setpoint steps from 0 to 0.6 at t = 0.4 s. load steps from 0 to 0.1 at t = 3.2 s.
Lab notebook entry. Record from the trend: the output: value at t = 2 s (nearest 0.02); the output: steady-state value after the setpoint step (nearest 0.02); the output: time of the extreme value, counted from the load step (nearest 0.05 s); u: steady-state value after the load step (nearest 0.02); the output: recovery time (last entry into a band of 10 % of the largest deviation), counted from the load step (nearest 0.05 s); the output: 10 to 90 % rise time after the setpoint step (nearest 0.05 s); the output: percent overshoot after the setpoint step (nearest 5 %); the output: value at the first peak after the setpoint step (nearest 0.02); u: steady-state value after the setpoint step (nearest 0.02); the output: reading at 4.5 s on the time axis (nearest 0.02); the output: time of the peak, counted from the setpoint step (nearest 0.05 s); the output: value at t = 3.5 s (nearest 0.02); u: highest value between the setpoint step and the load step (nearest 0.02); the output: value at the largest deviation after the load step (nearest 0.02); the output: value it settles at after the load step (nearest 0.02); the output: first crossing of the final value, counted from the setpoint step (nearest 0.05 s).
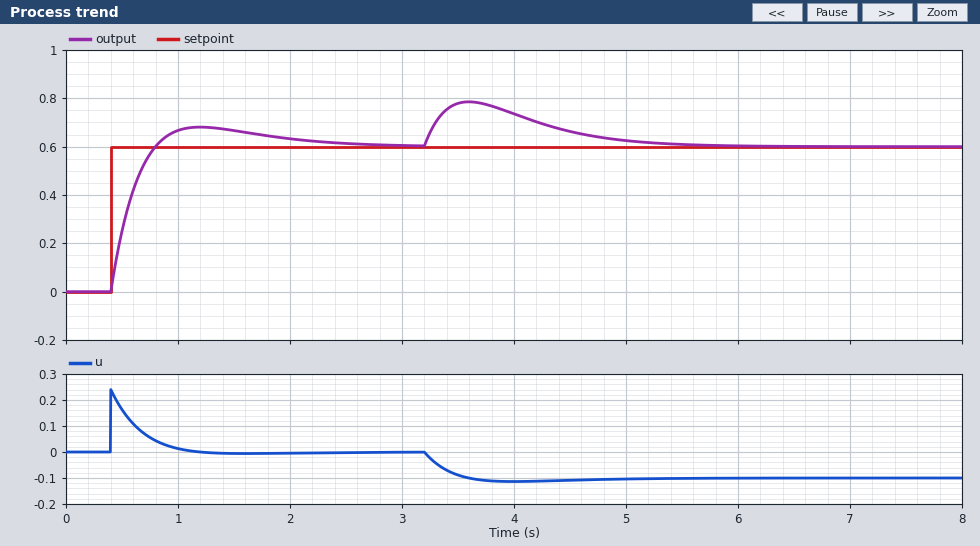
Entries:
0.64
0.60
0.40 s
-0.10
1.95 s
0.30 s
15 %
0.68
0.00
0.66
0.80 s
0.78
0.24
0.78
0.60
0.40 s
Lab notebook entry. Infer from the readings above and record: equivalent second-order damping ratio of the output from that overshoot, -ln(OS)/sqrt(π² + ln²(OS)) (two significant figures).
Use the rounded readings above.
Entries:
0.52
